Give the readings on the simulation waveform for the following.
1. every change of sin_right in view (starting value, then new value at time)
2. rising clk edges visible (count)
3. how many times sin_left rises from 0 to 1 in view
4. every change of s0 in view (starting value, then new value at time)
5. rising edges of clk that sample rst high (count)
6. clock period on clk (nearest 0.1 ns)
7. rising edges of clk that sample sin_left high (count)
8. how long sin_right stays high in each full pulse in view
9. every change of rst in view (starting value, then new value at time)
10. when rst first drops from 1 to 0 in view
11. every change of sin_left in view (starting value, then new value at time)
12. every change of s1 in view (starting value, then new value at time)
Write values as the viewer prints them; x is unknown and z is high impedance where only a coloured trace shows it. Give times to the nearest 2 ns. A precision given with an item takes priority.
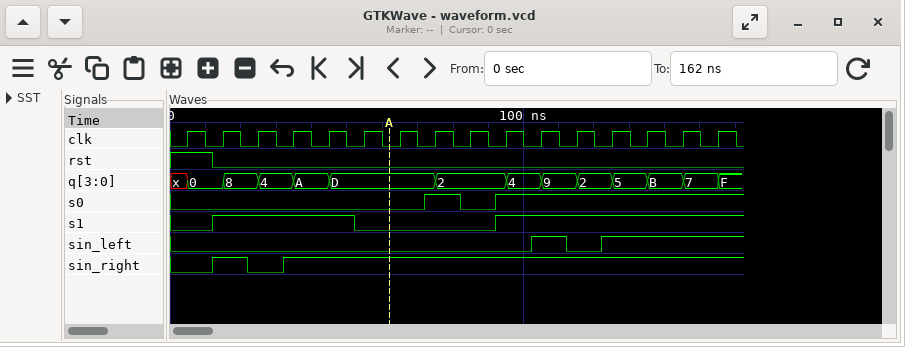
0, 1 at 12 ns, 0 at 22 ns, 1 at 32 ns
16
2
0, 1 at 72 ns, 0 at 82 ns, 1 at 92 ns
1
10 ns
5
10 ns
1, 0 at 12 ns
12 ns
0, 1 at 102 ns, 0 at 112 ns, 1 at 122 ns
0, 1 at 12 ns, 0 at 52 ns, 1 at 92 ns
